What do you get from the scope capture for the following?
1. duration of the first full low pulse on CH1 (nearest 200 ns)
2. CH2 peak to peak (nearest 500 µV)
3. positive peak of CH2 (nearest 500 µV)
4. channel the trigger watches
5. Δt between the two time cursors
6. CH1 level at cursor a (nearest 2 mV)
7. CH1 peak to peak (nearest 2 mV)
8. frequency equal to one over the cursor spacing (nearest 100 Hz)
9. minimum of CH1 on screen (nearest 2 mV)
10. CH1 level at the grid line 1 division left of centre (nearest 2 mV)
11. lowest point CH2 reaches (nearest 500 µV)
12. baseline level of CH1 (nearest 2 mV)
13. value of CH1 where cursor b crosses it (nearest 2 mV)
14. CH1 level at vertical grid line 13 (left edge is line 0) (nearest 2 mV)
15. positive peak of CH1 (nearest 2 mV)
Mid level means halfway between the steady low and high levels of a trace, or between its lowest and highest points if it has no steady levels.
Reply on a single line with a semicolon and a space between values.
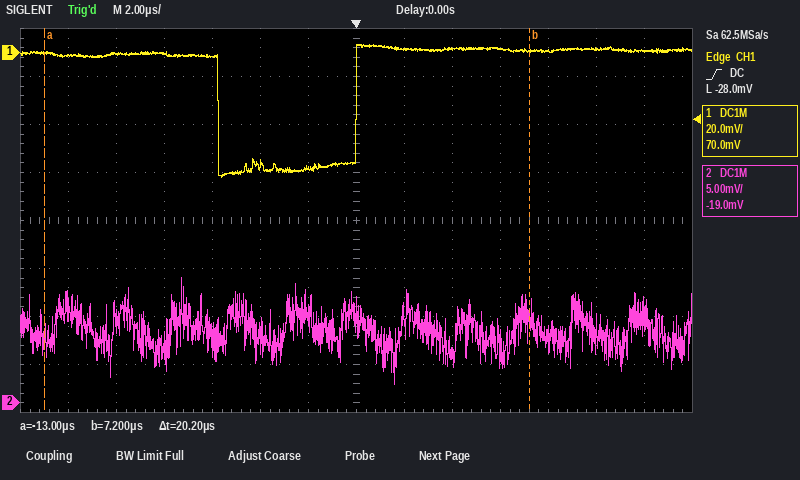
5.8 µs; 11.0 mV; 13.0 mV; CH1; 20.2 µs; 0 mV; 56 mV; 49.5 kHz; -52 mV; -48 mV; 2.0 mV; 0 mV; 0 mV; 0 mV; 4 mV
